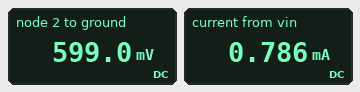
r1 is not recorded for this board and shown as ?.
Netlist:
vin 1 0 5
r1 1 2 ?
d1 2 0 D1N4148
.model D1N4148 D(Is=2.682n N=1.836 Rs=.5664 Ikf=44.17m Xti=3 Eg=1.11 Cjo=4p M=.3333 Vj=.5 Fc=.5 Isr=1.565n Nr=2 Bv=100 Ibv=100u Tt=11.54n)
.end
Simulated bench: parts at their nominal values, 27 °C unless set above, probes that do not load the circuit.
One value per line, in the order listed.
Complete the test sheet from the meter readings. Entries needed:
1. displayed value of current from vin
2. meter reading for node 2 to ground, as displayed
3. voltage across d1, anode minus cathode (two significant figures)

0.786 mA
599.0 mV
600 mV
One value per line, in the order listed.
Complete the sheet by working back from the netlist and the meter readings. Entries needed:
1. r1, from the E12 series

5.6 kΩ
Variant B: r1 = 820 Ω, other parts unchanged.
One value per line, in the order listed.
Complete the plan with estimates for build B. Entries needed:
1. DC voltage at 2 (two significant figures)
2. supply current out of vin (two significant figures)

700 mV
5.2 mA
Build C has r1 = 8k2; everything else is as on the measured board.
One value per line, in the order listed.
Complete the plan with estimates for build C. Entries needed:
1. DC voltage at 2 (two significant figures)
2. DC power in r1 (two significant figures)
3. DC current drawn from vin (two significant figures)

580 mV
2.4 mW
540 µA
